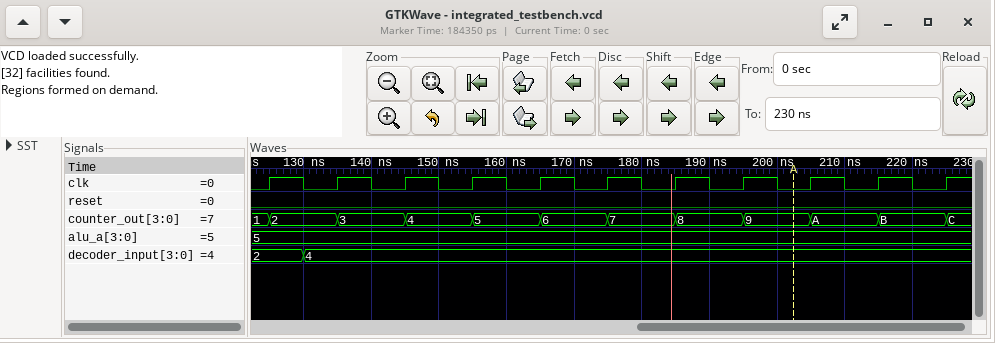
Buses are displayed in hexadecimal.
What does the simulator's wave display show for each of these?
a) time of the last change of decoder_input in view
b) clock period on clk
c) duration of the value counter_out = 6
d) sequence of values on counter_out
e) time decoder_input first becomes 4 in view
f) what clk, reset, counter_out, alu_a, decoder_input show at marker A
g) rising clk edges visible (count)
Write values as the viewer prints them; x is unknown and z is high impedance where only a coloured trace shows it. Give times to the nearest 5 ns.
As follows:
130 ns
10 ns
10 ns
1, 2, 3, 4, 5, 6, 7, 8, 9, A, B, C
130 ns
clk=0, reset=0, counter_out=9, alu_a=5, decoder_input=4
11
